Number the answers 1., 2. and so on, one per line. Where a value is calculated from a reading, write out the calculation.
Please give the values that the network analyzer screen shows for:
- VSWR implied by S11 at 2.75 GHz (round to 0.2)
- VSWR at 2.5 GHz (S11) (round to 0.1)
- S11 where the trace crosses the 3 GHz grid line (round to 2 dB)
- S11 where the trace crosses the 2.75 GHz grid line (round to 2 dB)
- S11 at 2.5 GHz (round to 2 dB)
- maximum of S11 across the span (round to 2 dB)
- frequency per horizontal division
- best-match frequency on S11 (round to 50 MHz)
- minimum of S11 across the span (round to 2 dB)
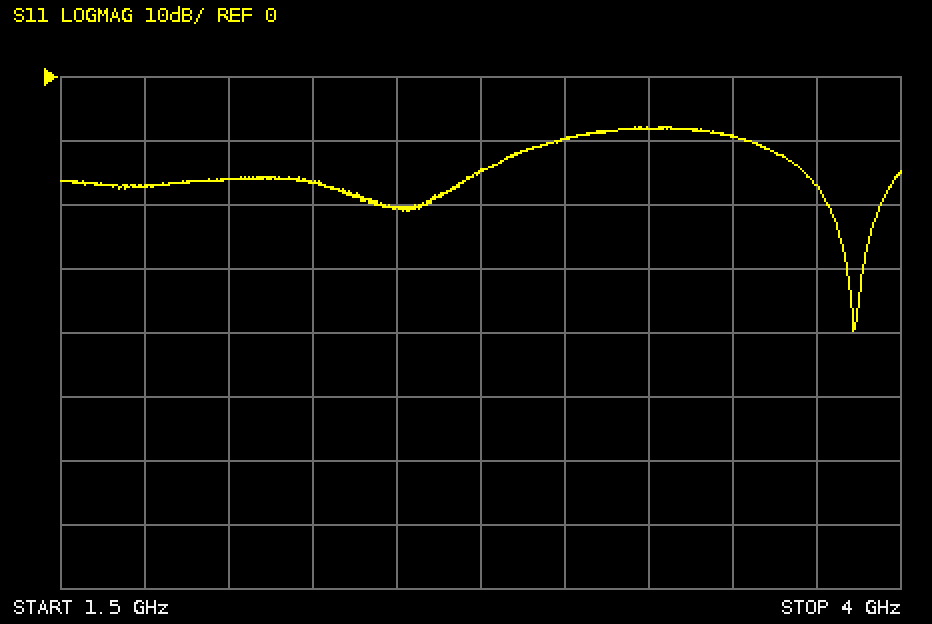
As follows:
1. |Γ| = 10^(-14/20) = 0.1995; VSWR = (1 + 0.1995)/(1 − 0.1995) ≈ 1.50, so 1.4 to the nearest 0.2
2. |Γ| = 10^(-20/20) = 0.1000; VSWR = (1 + 0.1000)/(1 − 0.1000) ≈ 1.2
3. -10 dB
4. -14 dB
5. -20 dB
6. -8 dB
7. 250 MHz
8. 3.85 GHz
9. -40 dB
